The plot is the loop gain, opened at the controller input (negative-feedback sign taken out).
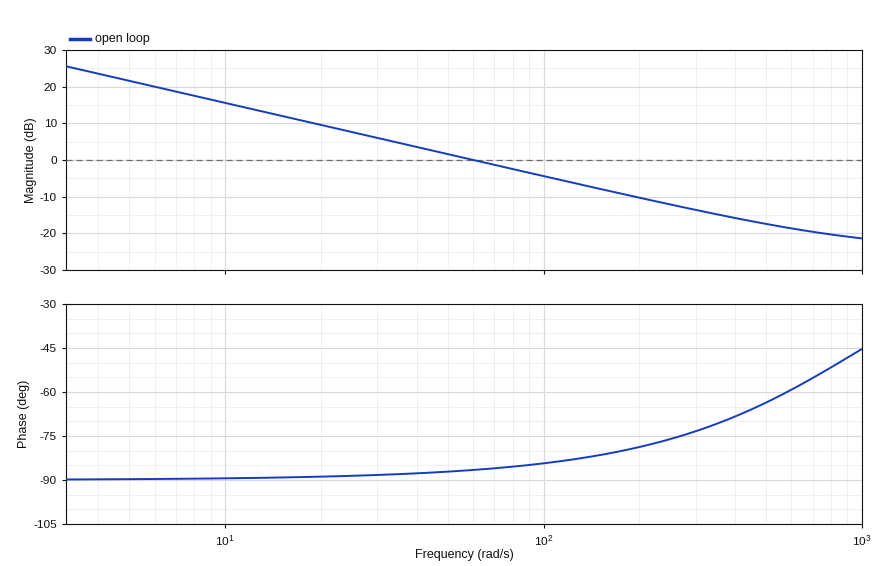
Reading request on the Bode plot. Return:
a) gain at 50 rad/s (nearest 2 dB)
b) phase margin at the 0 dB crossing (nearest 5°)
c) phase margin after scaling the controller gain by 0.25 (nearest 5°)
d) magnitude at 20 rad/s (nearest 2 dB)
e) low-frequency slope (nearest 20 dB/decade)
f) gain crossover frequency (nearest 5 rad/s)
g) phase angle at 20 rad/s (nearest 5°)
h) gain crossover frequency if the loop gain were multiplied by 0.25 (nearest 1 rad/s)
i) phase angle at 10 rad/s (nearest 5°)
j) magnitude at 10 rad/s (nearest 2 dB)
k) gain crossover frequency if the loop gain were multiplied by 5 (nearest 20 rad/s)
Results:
2 dB
95°
90°
10 dB
-20 dB/decade
60 rad/s
-90°
15 rad/s
-90°
16 dB
320 rad/s
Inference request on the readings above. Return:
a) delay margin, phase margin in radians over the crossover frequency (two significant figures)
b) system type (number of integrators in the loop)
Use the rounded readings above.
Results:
0.028 s
1
